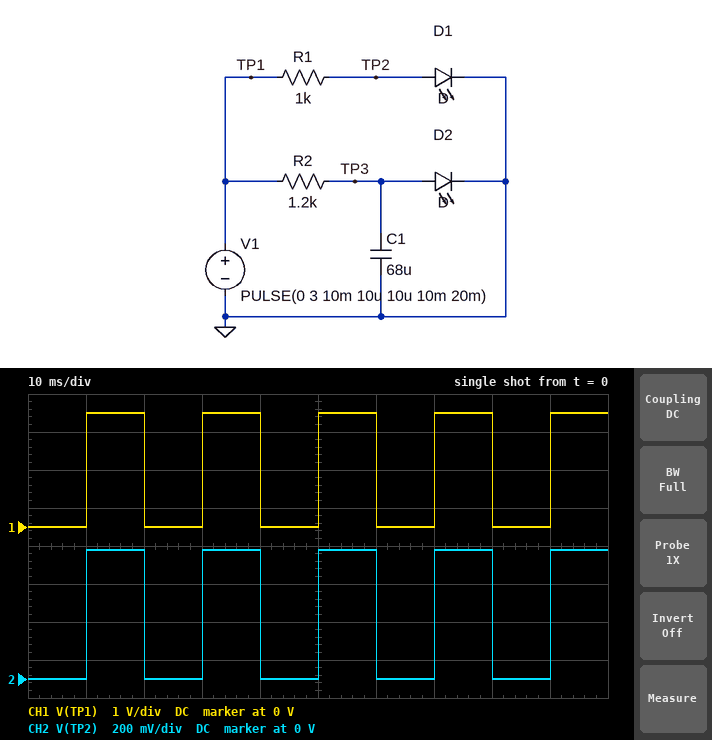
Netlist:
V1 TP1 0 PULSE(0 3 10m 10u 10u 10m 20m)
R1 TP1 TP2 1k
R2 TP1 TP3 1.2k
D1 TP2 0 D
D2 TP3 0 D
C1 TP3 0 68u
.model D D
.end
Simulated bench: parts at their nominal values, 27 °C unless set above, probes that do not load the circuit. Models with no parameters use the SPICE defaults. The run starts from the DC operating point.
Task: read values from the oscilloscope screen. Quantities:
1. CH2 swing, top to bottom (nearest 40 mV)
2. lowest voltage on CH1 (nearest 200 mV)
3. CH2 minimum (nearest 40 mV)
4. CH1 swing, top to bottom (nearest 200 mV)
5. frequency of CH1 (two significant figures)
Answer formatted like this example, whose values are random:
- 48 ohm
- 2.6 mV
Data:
- 680 mV
- 0 V
- 0 V
- 3.0 V
- 50 Hz
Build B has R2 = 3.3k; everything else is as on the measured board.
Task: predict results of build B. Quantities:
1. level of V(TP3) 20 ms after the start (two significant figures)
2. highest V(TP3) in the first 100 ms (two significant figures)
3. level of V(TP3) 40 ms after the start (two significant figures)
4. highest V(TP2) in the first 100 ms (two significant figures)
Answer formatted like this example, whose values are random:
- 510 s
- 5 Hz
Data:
- 130 mV
- 550 mV
- 250 mV
- 680 mV
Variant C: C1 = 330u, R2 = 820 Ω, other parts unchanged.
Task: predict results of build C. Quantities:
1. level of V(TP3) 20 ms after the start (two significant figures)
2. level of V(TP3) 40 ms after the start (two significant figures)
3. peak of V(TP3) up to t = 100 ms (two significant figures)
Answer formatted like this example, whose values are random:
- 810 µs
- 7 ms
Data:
- 110 mV
- 210 mV
- 470 mV
